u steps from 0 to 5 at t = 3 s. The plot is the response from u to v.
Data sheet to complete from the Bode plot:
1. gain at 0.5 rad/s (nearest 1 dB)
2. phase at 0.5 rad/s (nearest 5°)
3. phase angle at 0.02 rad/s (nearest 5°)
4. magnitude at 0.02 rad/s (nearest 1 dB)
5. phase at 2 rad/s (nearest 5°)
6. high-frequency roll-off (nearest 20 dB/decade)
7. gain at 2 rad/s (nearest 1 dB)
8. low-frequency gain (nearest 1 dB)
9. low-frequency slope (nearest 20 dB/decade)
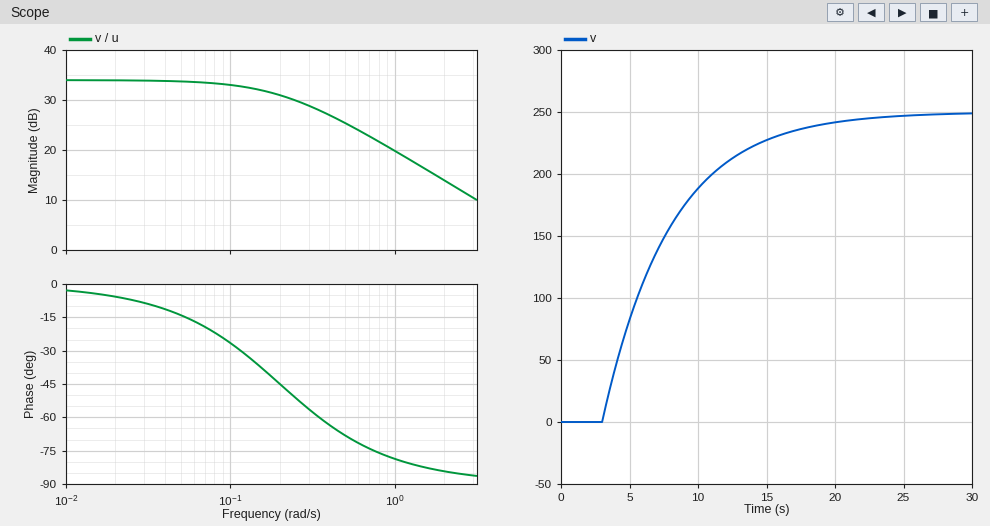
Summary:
25 dB
-70°
-5°
34 dB
-85°
-20 dB/decade
14 dB
34 dB
0 dB/decade
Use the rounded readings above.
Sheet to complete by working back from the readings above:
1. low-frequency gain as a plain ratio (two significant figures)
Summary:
50
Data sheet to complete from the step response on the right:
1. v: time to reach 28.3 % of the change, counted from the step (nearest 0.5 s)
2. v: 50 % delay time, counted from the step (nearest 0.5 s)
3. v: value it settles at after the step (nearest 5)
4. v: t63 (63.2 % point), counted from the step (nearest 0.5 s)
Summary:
1.5 s
3.5 s
250
5.0 s
